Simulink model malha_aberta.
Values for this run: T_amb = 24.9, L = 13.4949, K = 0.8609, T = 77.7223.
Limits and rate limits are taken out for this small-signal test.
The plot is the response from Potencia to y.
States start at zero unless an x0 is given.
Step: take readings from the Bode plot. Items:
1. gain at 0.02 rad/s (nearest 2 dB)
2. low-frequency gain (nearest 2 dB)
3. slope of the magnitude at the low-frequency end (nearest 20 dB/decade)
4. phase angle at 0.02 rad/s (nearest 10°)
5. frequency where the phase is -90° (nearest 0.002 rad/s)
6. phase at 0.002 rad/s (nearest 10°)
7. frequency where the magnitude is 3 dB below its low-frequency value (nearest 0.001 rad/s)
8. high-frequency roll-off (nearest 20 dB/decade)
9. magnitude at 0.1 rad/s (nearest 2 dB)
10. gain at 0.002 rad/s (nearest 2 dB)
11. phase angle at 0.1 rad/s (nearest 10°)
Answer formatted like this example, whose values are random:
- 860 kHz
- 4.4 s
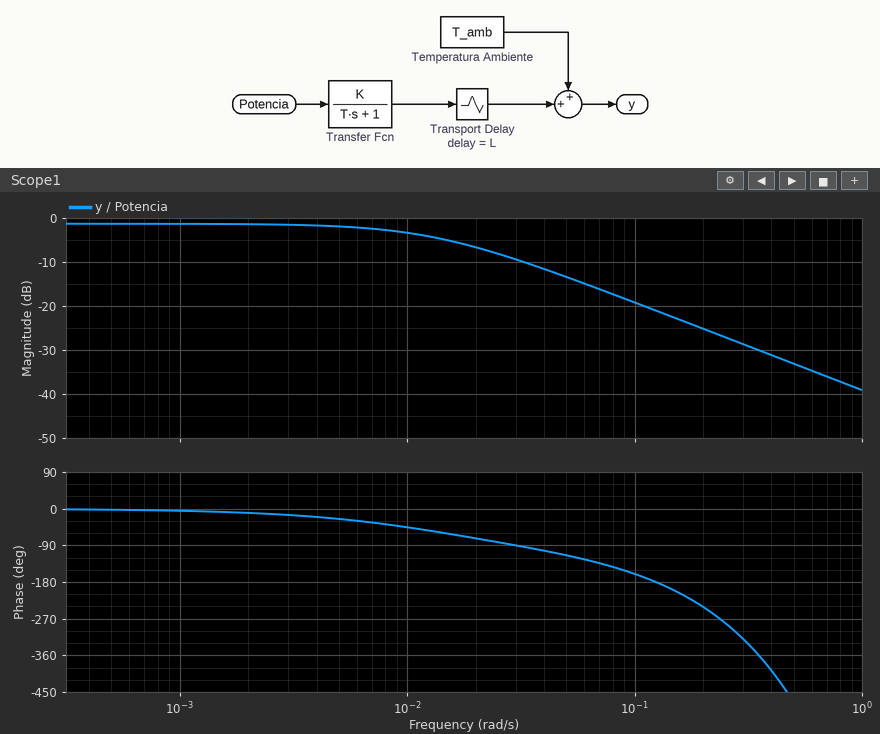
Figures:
- -6 dB
- -2 dB
- 0 dB/decade
- -70°
- 0.030 rad/s
- -10°
- 0.013 rad/s
- -20 dB/decade
- -20 dB
- -2 dB
- -160°
